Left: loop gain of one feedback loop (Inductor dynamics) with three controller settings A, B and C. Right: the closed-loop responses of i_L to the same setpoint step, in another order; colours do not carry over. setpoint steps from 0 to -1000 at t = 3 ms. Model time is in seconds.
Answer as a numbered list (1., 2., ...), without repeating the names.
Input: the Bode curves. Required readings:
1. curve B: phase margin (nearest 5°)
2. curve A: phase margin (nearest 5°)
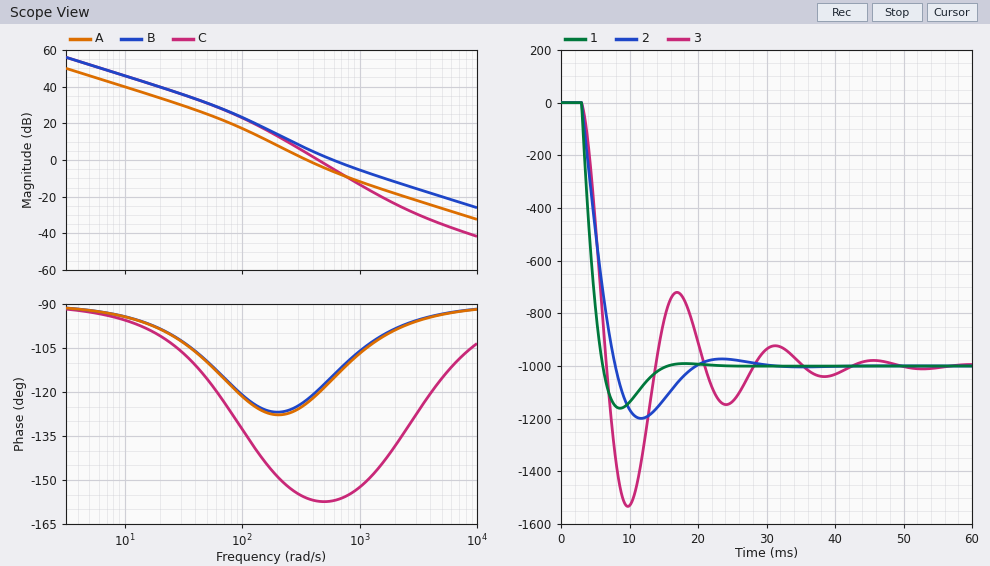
1. 65°
2. 55°
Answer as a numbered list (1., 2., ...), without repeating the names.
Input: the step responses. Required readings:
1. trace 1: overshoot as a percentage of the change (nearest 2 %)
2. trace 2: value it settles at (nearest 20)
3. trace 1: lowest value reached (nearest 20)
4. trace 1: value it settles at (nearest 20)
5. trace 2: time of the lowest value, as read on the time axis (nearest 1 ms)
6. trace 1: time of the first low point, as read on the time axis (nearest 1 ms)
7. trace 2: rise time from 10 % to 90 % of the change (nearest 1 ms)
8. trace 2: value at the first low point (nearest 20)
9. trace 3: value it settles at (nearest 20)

1. 16 %
2. -1000
3. -1160
4. -1000
5. 12 ms
6. 9 ms
7. 4 ms
8. -1200
9. -1000
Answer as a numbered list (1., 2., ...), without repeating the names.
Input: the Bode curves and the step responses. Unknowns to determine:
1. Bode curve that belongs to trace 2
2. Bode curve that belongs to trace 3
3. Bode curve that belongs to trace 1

1. A
2. C
3. B
